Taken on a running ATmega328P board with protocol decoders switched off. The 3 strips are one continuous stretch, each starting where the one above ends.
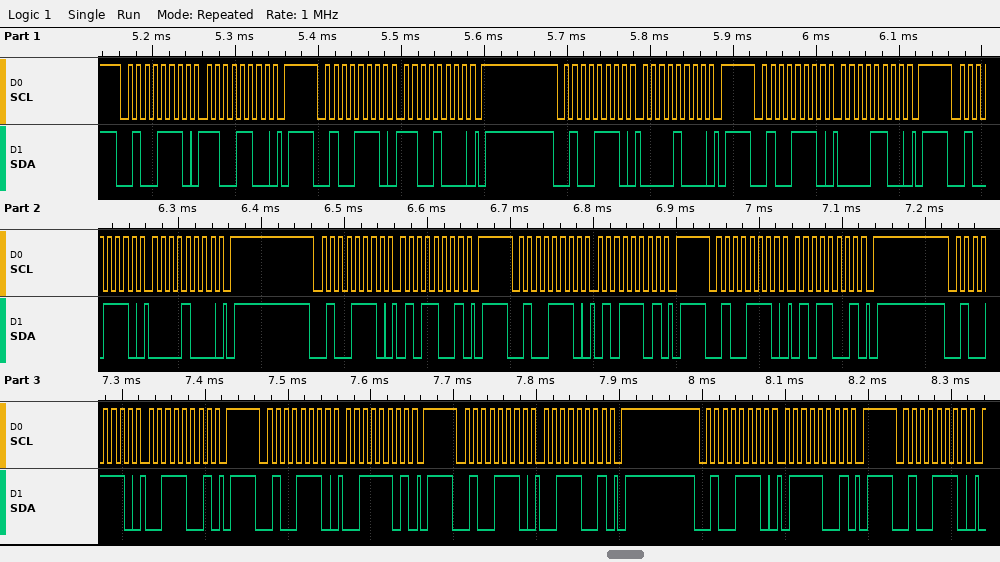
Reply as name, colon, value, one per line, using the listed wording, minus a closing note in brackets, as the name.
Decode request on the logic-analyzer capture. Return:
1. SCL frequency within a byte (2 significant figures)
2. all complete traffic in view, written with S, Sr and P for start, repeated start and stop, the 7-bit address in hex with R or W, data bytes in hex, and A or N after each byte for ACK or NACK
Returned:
SCL frequency within a byte: 100 kHz
all complete traffic in view, written with S, Sr and P for start, repeated start and stop, the 7-bit address in hex with R or W, data bytes in hex, and A or N after each byte for ACK or NACK: S 27W A CC A P S 27W A C8 A P S 27W A 08 A P S 27W A 0C A P S 27W A 08 A P S 27W A 59 A P S 27W A 5D A P S 27W A 59 A P S 27W A 39 A P S 27W A 3D A P S 27W A 39 A P S 27W A 79 A P S 27W A
